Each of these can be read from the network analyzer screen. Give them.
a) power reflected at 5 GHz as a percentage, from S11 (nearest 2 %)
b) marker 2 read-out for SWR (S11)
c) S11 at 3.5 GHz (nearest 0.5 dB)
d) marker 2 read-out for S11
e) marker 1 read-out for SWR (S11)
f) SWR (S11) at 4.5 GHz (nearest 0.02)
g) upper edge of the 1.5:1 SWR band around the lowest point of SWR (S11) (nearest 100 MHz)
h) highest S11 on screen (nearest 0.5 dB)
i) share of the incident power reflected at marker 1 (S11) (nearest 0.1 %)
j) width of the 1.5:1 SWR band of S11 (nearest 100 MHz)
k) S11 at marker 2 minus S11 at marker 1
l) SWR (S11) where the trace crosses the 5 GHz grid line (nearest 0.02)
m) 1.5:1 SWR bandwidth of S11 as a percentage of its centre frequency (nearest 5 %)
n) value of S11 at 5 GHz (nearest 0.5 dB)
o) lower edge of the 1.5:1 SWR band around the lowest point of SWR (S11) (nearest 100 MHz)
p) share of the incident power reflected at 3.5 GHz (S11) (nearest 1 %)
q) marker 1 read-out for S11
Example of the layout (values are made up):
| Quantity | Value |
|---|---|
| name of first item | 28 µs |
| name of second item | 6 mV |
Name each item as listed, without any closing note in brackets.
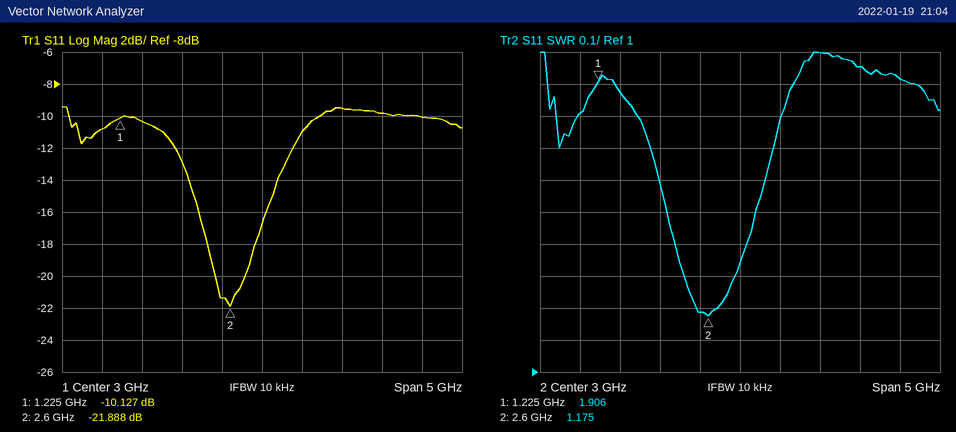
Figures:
| Quantity | Value |
|---|---|
| power reflected at 5 GHz as a percentage, from S11 | 10 % |
| marker 2 read-out for SWR | 1.175 |
| S11 at 3.5 GHz | -11.0 dB |
| marker 2 read-out for S11 | -21.888 dB |
| marker 1 read-out for SWR | 1.906 |
| SWR (S11) at 4.5 GHz | 1.96 |
| upper edge of the 1.5:1 SWR band around the lowest point of SWR (S11) | 3.2 GHz |
| highest S11 on screen | -9.5 dB |
| share of the incident power reflected at marker 1 (S11) | 9.7 % |
| width of the 1.5:1 SWR band of S11 | 1.1 GHz |
| S11 at marker 2 minus S11 at marker 1 | -11.761 dB |
| SWR (S11) where the trace crosses the 5 GHz grid line | 1.92 |
| 1.5:1 SWR bandwidth of S11 as a percentage of its centre frequency | 40 % |
| value of S11 at 5 GHz | -10.0 dB |
| lower edge of the 1.5:1 SWR band around the lowest point of SWR (S11) | 2.1 GHz |
| share of the incident power reflected at 3.5 GHz (S11) | 8 % |
| marker 1 read-out for S11 | -10.127 dB |
